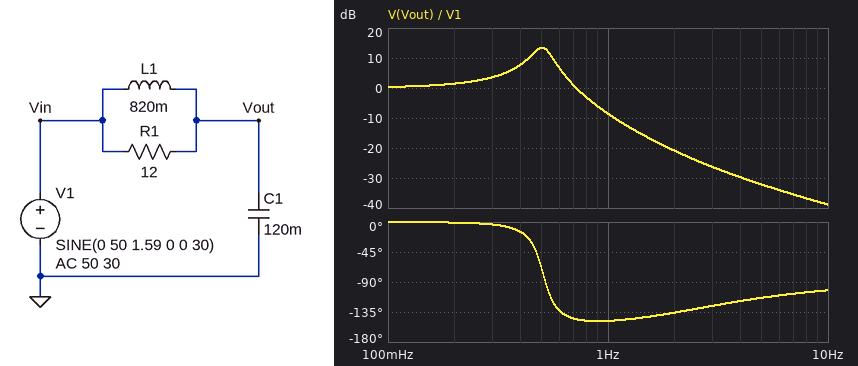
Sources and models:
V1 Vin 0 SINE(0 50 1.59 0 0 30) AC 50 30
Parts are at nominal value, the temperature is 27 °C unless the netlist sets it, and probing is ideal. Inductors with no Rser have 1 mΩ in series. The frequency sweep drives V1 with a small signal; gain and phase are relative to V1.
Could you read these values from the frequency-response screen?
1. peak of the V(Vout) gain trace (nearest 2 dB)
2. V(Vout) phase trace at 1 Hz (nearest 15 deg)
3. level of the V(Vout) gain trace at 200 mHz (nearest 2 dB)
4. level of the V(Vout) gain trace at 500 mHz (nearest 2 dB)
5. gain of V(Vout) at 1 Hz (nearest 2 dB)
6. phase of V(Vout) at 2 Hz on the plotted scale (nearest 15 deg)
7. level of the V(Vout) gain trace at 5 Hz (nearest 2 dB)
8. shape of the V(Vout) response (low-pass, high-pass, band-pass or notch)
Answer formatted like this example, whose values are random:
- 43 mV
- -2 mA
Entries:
- 14 dB
- -150 deg
- 2 dB
- 14 dB
- -8 dB
- -135 deg
- -32 dB
- low-pass
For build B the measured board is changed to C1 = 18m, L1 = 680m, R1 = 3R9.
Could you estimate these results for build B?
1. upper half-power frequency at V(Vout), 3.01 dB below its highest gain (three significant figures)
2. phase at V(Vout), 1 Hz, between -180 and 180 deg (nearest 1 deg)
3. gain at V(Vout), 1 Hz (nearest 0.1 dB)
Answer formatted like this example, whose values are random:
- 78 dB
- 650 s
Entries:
- 2.46 Hz
- -17 deg
- 1.8 dB
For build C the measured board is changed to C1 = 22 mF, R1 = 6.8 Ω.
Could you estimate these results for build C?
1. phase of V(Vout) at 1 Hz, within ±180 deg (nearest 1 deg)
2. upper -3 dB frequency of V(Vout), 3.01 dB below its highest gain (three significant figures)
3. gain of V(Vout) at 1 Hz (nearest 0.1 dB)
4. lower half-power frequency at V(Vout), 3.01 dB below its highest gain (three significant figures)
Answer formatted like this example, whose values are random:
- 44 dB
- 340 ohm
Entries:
- -32 deg
- 1.58 Hz
- 3.8 dB
- 366 mHz
